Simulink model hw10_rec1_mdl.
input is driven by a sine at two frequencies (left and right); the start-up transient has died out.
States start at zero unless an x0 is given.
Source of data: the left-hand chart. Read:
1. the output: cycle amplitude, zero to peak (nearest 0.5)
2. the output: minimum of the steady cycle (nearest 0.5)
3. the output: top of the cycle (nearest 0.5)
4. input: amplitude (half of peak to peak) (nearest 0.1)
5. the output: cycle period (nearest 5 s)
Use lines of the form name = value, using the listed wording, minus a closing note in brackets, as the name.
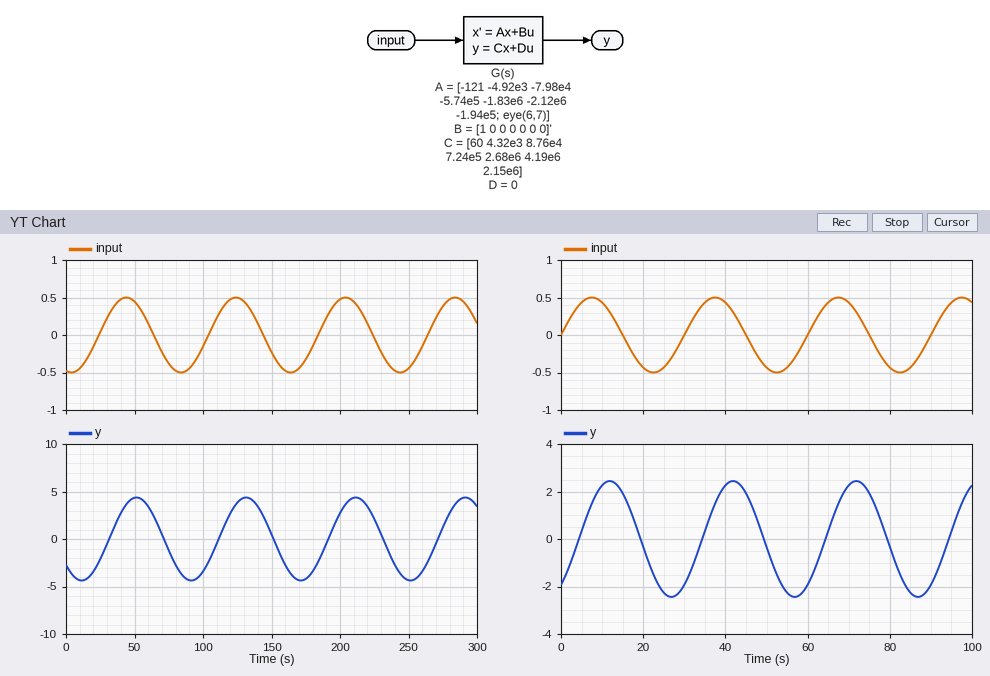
the output: cycle amplitude, zero to peak = 4.5
the output: minimum of the steady cycle = -4.5
the output: top of the cycle = 4.5
input: amplitude (half of peak to peak) = 0.5
the output: cycle period = 80 s
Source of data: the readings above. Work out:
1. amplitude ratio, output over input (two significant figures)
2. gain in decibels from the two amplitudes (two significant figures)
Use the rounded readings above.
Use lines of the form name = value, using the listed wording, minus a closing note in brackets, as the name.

amplitude ratio, output over input = 9.0
gain in decibels from the two amplitudes = 19 dB
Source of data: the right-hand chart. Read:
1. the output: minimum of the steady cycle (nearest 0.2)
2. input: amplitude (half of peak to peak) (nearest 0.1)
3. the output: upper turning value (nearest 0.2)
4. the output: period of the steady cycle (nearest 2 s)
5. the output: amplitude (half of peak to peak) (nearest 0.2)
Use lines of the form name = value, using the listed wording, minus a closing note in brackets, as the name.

the output: minimum of the steady cycle = -2.4
input: amplitude (half of peak to peak) = 0.5
the output: upper turning value = 2.4
the output: period of the steady cycle = 30 s
the output: amplitude (half of peak to peak) = 2.4
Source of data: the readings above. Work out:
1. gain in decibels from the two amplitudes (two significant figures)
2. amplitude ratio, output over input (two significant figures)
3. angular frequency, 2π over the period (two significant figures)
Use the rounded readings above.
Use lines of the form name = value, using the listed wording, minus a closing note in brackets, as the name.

gain in decibels from the two amplitudes = 14 dB
amplitude ratio, output over input = 4.8
angular frequency, 2π over the period = 0.21 rad/s
